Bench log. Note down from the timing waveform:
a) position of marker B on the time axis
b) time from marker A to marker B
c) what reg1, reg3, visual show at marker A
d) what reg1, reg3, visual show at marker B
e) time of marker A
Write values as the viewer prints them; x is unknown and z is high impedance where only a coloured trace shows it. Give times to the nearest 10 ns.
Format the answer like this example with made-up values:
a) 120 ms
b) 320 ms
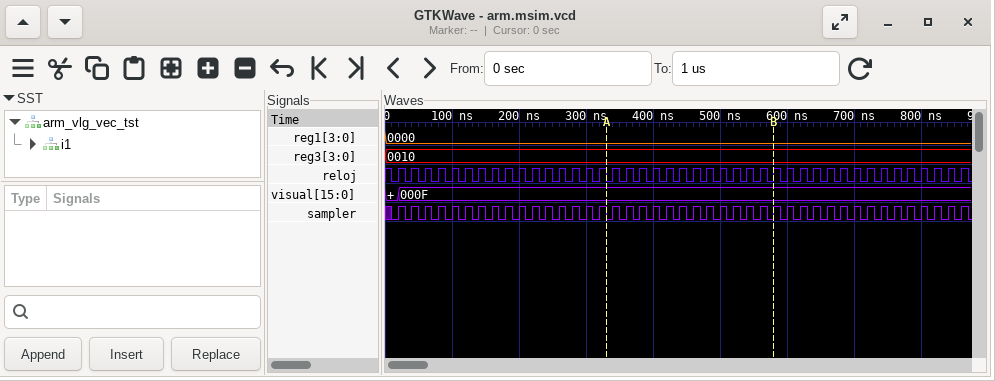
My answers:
a) 580 ns
b) 250 ns
c) reg1=0000, reg3=0010, visual=000F
d) reg1=0000, reg3=0010, visual=000F
e) 330 ns
